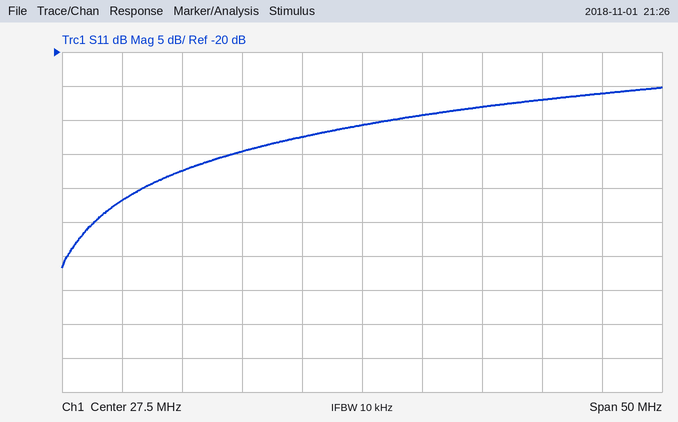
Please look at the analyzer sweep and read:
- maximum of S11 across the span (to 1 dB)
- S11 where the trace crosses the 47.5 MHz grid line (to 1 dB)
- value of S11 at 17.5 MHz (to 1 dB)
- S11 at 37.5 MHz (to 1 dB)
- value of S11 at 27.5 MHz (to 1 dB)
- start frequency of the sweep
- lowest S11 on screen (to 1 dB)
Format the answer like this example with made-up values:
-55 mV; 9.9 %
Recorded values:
-25 dB; -26 dB; -35 dB; -28 dB; -31 dB; 2.5 MHz; -52 dB
